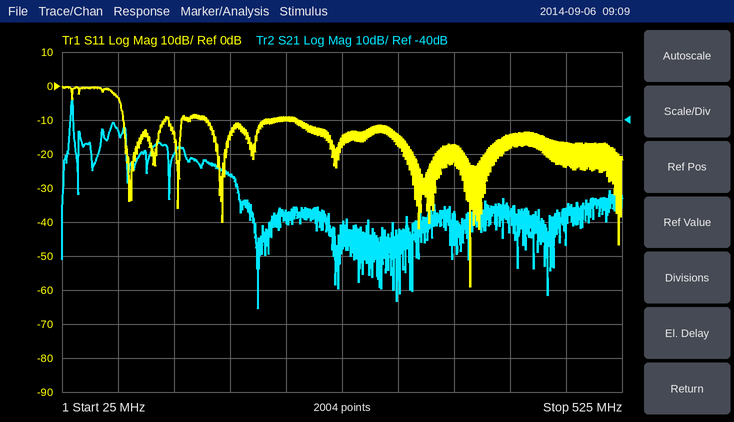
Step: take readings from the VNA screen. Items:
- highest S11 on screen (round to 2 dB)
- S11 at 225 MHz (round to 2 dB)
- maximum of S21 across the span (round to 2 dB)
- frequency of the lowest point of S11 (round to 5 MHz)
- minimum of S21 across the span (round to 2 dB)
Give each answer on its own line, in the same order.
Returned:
0 dB
-10 dB
-34 dB
390 MHz
-96 dB
